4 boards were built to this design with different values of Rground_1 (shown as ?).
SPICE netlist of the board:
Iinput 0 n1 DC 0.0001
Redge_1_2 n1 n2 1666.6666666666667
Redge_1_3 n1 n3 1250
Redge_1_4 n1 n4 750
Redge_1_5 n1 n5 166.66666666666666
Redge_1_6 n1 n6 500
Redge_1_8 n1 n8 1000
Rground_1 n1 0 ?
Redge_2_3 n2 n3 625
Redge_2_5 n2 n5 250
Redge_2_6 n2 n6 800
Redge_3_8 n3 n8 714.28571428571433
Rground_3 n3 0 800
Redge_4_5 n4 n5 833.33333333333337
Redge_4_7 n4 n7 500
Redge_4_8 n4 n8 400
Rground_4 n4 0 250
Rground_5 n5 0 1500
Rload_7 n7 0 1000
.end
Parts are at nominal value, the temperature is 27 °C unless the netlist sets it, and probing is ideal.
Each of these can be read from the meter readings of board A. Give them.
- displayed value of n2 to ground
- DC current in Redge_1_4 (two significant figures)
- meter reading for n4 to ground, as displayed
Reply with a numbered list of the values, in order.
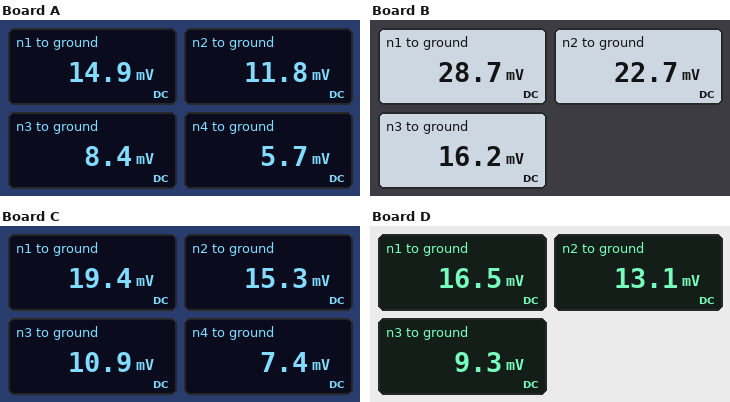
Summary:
1. 11.8 mV
2. 12 µA
3. 5.7 mV
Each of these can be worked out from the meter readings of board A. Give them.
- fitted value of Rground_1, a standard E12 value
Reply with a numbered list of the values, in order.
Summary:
1. 270 Ω
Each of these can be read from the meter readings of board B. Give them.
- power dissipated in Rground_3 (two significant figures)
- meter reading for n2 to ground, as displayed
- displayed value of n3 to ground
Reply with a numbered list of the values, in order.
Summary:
1. 330 nW
2. 22.7 mV
3. 16.2 mV
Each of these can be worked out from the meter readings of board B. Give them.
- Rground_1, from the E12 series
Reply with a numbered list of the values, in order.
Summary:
1. 2.2 kΩ
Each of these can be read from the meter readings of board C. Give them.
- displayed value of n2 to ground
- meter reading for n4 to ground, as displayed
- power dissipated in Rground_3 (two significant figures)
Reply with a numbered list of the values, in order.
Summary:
1. 15.3 mV
2. 7.4 mV
3. 150 nW
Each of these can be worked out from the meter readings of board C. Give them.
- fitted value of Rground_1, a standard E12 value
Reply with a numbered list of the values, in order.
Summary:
1. 470 Ω
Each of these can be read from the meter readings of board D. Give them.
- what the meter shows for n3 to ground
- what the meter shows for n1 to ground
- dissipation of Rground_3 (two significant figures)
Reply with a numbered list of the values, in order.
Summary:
1. 9.3 mV
2. 16.5 mV
3. 110 nW
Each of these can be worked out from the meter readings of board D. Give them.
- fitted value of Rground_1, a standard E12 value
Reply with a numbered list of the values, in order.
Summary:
1. 330 Ω
